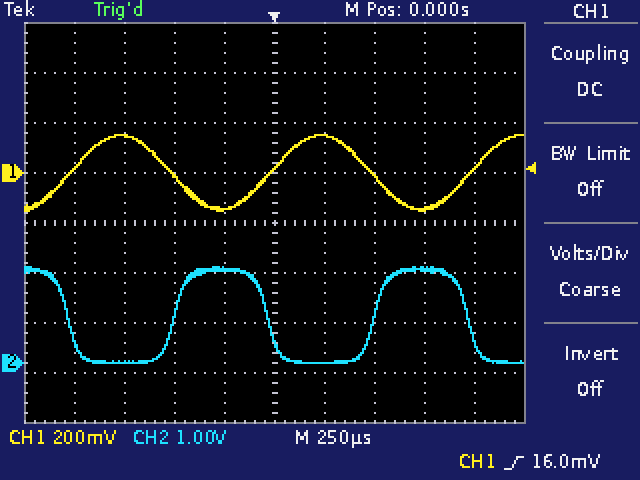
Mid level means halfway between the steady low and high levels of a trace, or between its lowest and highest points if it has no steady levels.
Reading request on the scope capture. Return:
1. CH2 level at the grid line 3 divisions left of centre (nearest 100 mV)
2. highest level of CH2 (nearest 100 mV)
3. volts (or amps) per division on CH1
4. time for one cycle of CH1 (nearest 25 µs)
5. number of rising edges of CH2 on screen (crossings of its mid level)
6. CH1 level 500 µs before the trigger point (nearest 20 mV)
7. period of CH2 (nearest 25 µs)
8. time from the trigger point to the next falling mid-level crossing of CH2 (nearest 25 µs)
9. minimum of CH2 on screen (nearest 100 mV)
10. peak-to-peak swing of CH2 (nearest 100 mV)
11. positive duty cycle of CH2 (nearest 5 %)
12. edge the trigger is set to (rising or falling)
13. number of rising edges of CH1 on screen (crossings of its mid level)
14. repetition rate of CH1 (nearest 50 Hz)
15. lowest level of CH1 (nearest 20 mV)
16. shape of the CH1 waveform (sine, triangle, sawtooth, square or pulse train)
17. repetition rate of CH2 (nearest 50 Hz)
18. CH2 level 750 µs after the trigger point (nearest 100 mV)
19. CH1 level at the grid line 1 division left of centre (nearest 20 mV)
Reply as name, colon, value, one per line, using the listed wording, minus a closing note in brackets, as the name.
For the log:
CH2 level at the grid line 3 divisions left of centre: 0.0 V
highest level of CH2: 1.9 V
volts (or amps) per division on CH1: 200 mV
time for one cycle of CH1: 1.000 ms
number of rising edges of CH2 on screen: 2
CH1 level 500 µs before the trigger point: -20 mV
period of CH2: 1.000 ms
time from the trigger point to the next falling mid-level crossing of CH2: 975 µs
minimum of CH2 on screen: 0.0 V
peak-to-peak swing of CH2: 1.9 V
positive duty cycle of CH2: 45 %
edge the trigger is set to: rising
number of rising edges of CH1 on screen: 3
repetition rate of CH1: 1.00 kHz
lowest level of CH1: -160 mV
shape of the CH1 waveform: sine
repetition rate of CH2: 1.00 kHz
CH2 level 750 µs after the trigger point: 1.9 V
CH1 level at the grid line 1 division left of centre: -140 mV
